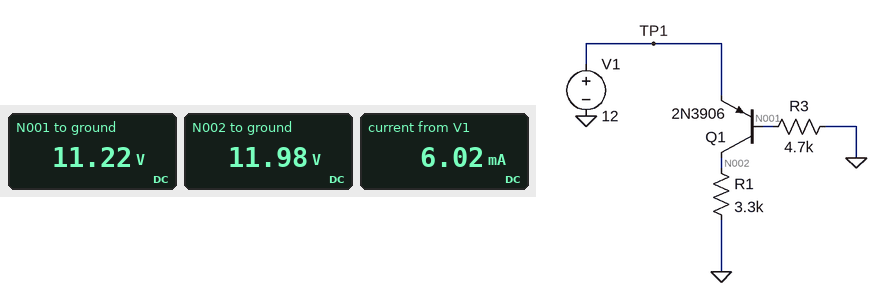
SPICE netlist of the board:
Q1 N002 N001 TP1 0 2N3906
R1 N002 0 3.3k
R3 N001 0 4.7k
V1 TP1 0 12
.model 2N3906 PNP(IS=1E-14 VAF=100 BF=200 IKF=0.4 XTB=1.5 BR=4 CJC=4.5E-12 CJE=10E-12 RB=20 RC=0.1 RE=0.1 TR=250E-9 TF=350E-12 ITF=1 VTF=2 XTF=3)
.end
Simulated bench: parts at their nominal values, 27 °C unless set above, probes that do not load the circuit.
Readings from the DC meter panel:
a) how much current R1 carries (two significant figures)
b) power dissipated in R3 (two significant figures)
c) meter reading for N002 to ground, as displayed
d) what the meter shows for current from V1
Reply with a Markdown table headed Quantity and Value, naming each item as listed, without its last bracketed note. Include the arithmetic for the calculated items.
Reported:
| Quantity | Value |
|---|---|
| how much current R1 carries | (11.98 V) / 3.3 kΩ = 3.6 mA |
| power dissipated in R3 | (11.22 V)^2 / 4.7 kΩ = 27 mW |
| meter reading for N002 to ground, as displayed | 11.98 V |
| what the meter shows for current from V1 | 6.02 mA |
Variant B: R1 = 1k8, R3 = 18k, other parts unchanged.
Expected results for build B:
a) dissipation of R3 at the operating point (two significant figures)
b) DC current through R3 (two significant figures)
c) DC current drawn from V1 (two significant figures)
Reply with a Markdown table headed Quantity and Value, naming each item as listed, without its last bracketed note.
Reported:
| Quantity | Value |
|---|---|
| dissipation of R3 at the operating point | 7.1 mW |
| DC current through R3 | 630 µA |
| DC current drawn from V1 | 7.3 mA |
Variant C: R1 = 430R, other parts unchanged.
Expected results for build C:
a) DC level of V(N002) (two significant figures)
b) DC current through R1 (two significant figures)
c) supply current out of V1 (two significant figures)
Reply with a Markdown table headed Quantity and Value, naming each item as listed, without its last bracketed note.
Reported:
| Quantity | Value |
|---|---|
| DC level of V(N002) | 12 V |
| DC current through R1 | 28 mA |
| supply current out of V1 | 30 mA |
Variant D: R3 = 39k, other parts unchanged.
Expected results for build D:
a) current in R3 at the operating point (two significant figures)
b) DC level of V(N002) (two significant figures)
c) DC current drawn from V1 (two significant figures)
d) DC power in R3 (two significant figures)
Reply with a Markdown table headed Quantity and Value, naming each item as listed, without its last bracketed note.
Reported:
| Quantity | Value |
|---|---|
| current in R3 at the operating point | 290 µA |
| DC level of V(N002) | 12 V |
| DC current drawn from V1 | 3.9 mA |
| DC power in R3 | 3.3 mW |
